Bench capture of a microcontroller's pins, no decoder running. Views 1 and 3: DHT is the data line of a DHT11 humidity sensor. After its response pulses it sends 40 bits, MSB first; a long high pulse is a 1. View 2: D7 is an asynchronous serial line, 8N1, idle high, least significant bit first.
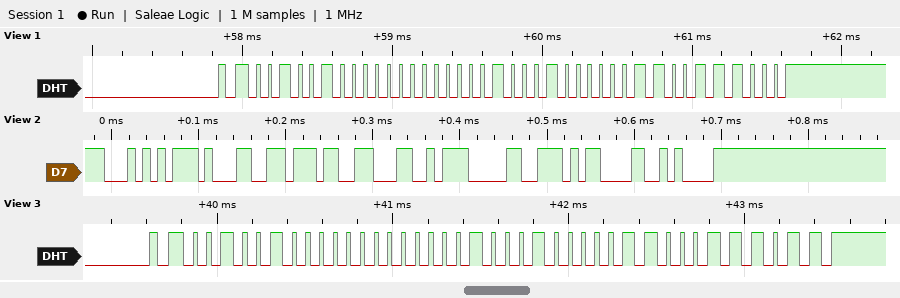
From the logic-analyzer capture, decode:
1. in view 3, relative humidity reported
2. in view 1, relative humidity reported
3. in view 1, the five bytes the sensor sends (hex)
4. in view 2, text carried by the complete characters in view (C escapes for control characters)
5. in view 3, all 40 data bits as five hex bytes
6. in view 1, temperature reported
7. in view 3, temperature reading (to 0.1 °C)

36 %
36 %
24 00 11 03 38
"T17L0\r\n"
24 00 11 06 3B
17.3 °C
17.6 °C
